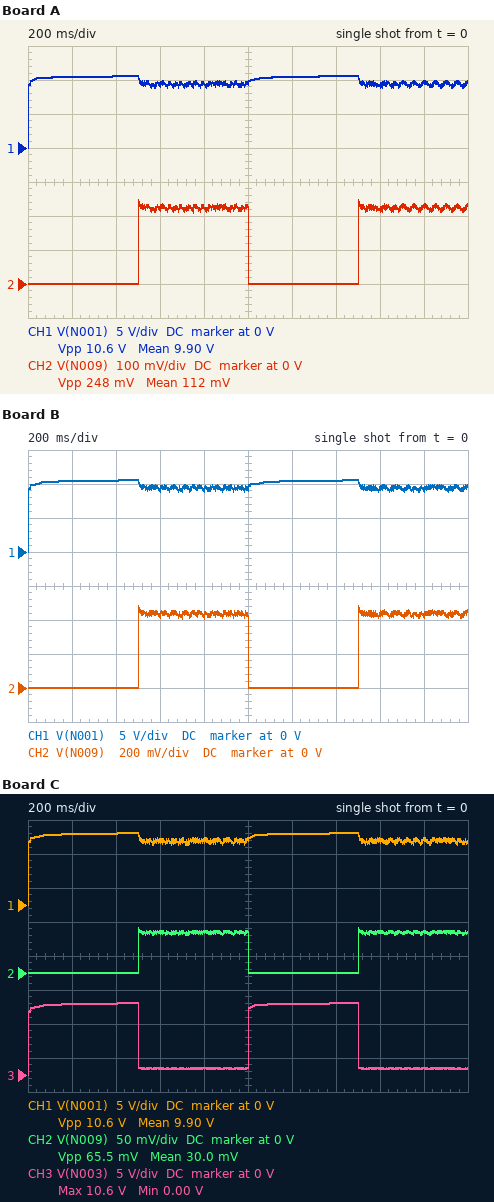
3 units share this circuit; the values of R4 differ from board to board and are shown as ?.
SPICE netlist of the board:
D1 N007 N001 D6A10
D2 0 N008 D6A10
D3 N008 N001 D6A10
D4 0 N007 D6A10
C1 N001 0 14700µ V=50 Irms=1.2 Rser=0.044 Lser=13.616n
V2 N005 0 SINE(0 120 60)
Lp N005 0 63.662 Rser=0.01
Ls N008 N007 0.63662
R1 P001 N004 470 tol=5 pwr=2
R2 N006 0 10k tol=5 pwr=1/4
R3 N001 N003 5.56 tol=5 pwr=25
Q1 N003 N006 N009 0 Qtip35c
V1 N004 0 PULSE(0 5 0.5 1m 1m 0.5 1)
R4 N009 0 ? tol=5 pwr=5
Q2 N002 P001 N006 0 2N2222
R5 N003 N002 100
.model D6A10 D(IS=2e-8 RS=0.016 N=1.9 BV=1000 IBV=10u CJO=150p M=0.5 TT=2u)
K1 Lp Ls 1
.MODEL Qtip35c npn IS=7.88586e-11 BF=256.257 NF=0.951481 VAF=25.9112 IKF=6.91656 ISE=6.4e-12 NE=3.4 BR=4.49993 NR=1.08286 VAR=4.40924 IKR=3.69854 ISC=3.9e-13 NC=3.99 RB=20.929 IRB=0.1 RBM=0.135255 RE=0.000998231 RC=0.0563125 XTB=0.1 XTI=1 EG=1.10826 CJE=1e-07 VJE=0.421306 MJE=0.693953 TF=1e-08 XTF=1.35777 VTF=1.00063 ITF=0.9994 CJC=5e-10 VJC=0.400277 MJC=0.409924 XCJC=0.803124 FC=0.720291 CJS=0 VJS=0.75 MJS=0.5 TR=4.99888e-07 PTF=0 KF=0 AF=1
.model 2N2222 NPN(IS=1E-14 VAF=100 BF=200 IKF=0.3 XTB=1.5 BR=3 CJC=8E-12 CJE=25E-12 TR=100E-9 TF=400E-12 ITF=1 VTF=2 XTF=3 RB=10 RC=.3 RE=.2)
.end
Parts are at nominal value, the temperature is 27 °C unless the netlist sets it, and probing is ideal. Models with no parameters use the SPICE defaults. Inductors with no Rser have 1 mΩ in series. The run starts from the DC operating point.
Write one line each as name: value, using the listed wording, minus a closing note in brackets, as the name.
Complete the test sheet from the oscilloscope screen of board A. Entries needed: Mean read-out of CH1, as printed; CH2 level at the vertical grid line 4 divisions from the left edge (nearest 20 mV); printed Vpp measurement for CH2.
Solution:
Mean read-out of CH1, as printed: 9.90 V
CH2 level at the vertical grid line 4 divisions from the left edge: 220 mV
printed Vpp measurement for CH2: 248 mV
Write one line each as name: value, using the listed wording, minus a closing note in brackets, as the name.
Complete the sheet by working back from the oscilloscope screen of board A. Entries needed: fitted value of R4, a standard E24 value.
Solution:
fitted value of R4, a standard E24 value: 0.15 Ω
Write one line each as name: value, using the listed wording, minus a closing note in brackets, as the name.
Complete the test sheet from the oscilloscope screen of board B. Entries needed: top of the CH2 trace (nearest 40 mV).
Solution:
top of the CH2 trace: 480 mV
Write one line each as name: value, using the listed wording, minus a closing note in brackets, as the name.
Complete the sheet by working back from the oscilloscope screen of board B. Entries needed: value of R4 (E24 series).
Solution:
value of R4: 0.3 Ω
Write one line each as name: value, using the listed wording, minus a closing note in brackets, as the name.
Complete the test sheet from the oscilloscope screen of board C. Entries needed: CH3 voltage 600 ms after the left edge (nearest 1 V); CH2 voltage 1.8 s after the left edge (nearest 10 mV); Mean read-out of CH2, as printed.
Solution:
CH3 voltage 600 ms after the left edge: 1 V
CH2 voltage 1.8 s after the left edge: 60 mV
Mean read-out of CH2, as printed: 30.0 mV
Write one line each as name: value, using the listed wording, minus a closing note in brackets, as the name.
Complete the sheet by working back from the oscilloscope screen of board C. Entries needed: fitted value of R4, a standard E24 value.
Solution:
fitted value of R4, a standard E24 value: 0.039 Ω
